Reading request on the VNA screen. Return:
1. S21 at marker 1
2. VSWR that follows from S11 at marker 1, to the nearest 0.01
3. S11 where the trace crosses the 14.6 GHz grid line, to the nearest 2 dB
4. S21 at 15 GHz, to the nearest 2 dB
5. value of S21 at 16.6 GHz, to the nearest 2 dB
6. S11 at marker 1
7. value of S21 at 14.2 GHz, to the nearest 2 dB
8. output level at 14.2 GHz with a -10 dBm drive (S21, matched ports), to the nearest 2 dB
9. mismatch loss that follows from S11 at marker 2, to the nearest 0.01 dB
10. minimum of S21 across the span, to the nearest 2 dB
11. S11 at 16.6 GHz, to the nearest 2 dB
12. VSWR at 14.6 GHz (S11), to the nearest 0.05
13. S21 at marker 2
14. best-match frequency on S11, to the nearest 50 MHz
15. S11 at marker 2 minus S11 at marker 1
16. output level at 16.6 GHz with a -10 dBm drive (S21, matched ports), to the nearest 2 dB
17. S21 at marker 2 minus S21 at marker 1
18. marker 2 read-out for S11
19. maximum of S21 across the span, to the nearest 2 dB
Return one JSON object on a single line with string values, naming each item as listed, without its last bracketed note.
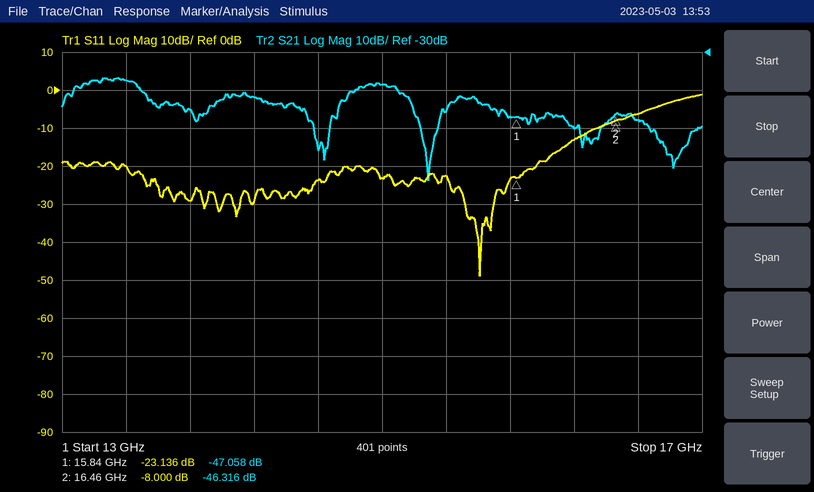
{"S21 at marker 1": "-47.058 dB", "VSWR that follows from S11 at marker 1, to the nearest 0.01": "1.15", "S11 where the trace crosses the 14.6 GHz grid line, to the nearest 2 dB": "-24 dB", "S21 at 15 GHz, to the nearest 2 dB": "-38 dB", "value of S21 at 16.6 GHz, to the nearest 2 dB": "-48 dB", "S11 at marker 1": "-23.136 dB", "value of S21 at 14.2 GHz, to the nearest 2 dB": "-42 dB", "output level at 14.2 GHz with a -10 dBm drive (S21, matched ports), to the nearest 2 dB": "-52 dBm", "mismatch loss that follows from S11 at marker 2, to the nearest 0.01 dB": "0.75 dB", "minimum of S21 across the span, to the nearest 2 dB": "-64 dB", "S11 at 16.6 GHz, to the nearest 2 dB": "-6 dB", "VSWR at 14.6 GHz (S11), to the nearest 0.05": "1.15", "S21 at marker 2": "-46.316 dB", "best-match frequency on S11, to the nearest 50 MHz": "15.60 GHz", "S11 at marker 2 minus S11 at marker 1": "15.136 dB", "output level at 16.6 GHz with a -10 dBm drive (S21, matched ports), to the nearest 2 dB": "-58 dBm", "S21 at marker 2 minus S21 at marker 1": "0.742 dB", "marker 2 read-out for S11": "-8.000 dB", "maximum of S21 across the span, to the nearest 2 dB": "-36 dB"}
